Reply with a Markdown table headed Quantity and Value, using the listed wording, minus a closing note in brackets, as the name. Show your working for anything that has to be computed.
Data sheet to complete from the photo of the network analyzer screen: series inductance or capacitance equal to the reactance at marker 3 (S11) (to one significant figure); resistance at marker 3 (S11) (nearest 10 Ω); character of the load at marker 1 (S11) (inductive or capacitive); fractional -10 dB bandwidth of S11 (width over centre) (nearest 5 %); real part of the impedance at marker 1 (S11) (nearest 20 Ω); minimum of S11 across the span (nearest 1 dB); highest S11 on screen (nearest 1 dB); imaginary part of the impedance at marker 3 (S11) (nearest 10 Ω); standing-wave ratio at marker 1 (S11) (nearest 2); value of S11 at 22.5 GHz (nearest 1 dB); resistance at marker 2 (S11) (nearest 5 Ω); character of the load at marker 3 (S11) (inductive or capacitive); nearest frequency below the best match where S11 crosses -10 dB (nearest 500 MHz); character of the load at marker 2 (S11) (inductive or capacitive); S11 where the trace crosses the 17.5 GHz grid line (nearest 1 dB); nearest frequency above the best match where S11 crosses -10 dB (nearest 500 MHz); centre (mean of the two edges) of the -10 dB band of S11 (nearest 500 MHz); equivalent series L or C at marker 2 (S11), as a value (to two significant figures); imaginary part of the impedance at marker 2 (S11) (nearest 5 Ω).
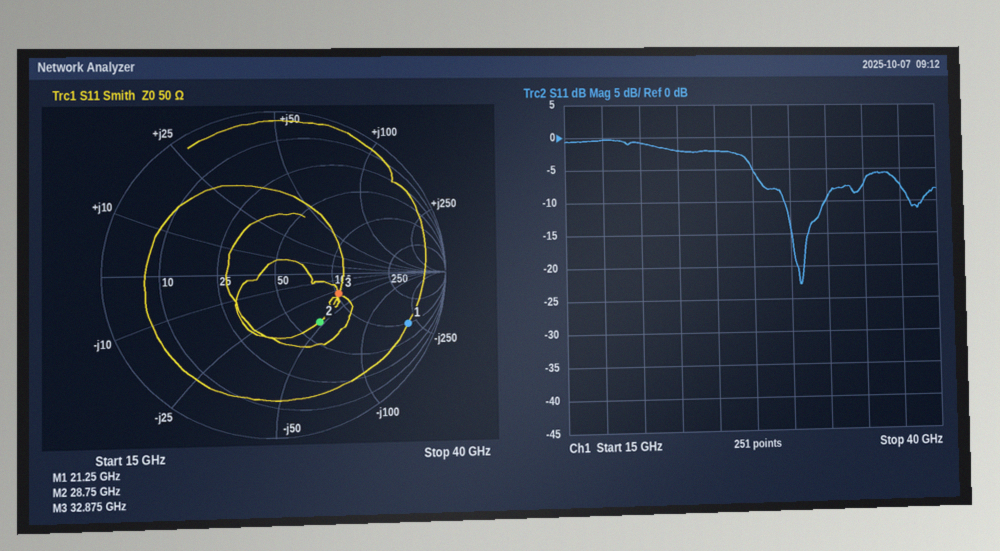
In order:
| Quantity | Value |
|---|---|
| series inductance or capacitance equal to the reactance at marker 3 (S11) | C = 1/(2π × 32.875 GHz × 30 Ω) ≈ 161 fF, so 200 fF to one significant figure |
| resistance at marker 3 (S11) | 100 Ω |
| character of the load at marker 1 (S11) | capacitive |
| fractional -10 dB bandwidth of S11 (width over centre) | 3 GHz / 31 GHz ≈ 10 % |
| real part of the impedance at marker 1 (S11) | 100 Ω |
| minimum of S11 across the span | -23 dB |
| highest S11 on screen | 0 dB |
| imaginary part of the impedance at marker 3 (S11) | -30 Ω |
| standing-wave ratio at marker 1 (S11) | 12 |
| value of S11 at 22.5 GHz | -2 dB |
| resistance at marker 2 (S11) | 65 Ω |
| character of the load at marker 3 (S11) | capacitive |
| nearest frequency below the best match where S11 crosses -10 dB | 29.5 GHz |
| character of the load at marker 2 (S11) | capacitive |
| S11 where the trace crosses the 17.5 GHz grid line | 0 dB |
| nearest frequency above the best match where S11 crosses -10 dB | 32.5 GHz |
| centre (mean of the two edges) of the -10 dB band of S11 | 31.0 GHz |
| equivalent series L or C at marker 2 (S11), as a value | C = 1/(2π × 28.75 GHz × 45 Ω) ≈ 123 fF, so 120 fF to two significant figures |
| imaginary part of the impedance at marker 2 (S11) | -45 Ω |
